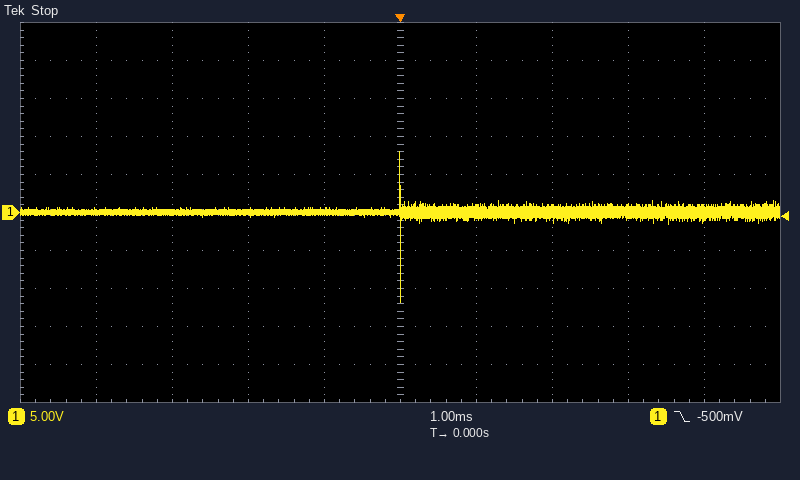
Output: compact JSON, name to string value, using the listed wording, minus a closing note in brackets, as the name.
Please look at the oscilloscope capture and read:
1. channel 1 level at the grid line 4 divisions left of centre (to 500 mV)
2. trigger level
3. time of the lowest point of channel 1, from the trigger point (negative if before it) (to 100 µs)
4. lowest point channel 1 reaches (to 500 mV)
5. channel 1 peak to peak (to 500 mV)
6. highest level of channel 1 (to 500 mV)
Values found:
{"channel 1 level at the grid line 4 divisions left of centre": "0.0 V", "trigger level": "-500 mV", "time of the lowest point of channel 1, from the trigger point (negative if before it)": "0.0 ms", "lowest point channel 1 reaches": "-12.0 V", "channel 1 peak to peak": "20.0 V", "highest level of channel 1": "8.0 V"}
